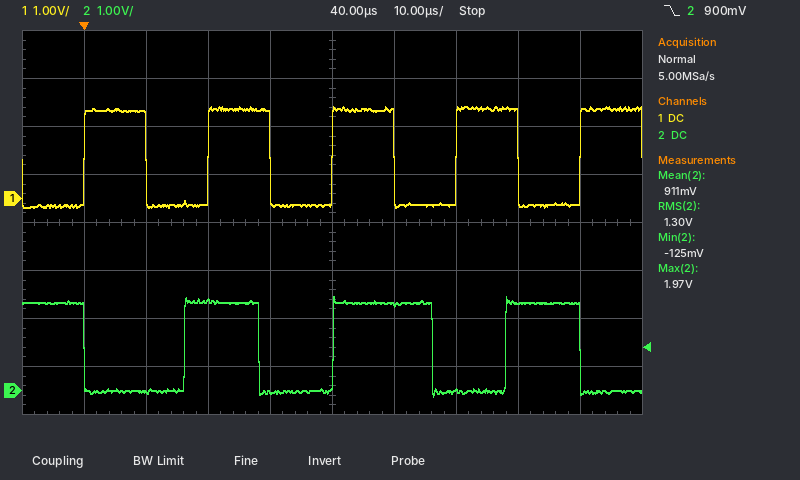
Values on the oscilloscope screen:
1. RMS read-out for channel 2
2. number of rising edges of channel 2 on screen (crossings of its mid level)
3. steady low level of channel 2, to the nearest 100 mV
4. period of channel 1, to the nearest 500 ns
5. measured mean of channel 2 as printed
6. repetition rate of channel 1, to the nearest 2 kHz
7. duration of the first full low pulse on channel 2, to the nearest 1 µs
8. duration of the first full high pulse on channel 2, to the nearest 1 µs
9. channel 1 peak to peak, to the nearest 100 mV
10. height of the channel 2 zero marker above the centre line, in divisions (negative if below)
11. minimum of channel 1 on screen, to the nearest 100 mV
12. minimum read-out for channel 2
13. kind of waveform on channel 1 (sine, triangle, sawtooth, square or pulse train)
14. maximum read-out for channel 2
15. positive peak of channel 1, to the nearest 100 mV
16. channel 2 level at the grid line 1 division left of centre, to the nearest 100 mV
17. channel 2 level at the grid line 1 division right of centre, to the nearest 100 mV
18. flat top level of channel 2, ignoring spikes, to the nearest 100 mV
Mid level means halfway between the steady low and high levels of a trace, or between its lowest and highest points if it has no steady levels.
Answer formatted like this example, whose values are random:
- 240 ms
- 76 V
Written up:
- 1.30 V
- 3
- 0.0 V
- 20.0 µs
- 911 mV
- 50 kHz
- 16 µs
- 12 µs
- 2.1 V
- -3.5 div
- -200 mV
- -125 mV
- square
- 1.97 V
- 1.9 V
- 0.0 V
- 1.8 V
- 1.8 V
